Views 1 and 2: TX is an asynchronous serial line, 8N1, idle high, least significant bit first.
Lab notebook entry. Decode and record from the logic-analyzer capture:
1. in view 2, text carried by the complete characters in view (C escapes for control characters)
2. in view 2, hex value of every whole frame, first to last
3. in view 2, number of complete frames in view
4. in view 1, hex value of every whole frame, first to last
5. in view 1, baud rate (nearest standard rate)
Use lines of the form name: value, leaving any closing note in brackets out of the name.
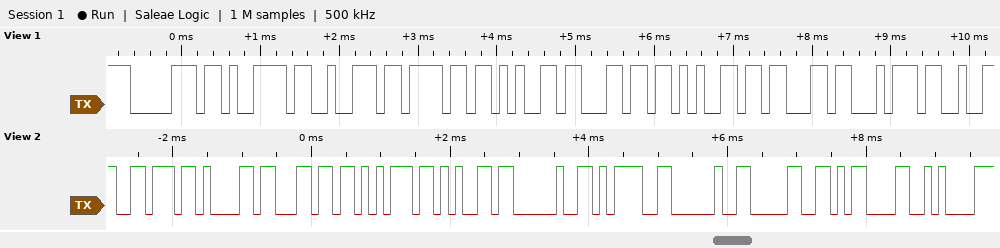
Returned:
in view 2, text carried by the complete characters in view: "value = 0\r\n"
in view 2, hex value of every whole frame, first to last: 0x76 0x61 0x6C 0x75 0x65 0x20 0x3D 0x20 0x30 0x0D 0x0A
in view 2, number of complete frames in view: 11
in view 1, hex value of every whole frame, first to last: 70 79 72 6F 65 6C 65 63 74
in view 1, baud rate: 9600 baud
